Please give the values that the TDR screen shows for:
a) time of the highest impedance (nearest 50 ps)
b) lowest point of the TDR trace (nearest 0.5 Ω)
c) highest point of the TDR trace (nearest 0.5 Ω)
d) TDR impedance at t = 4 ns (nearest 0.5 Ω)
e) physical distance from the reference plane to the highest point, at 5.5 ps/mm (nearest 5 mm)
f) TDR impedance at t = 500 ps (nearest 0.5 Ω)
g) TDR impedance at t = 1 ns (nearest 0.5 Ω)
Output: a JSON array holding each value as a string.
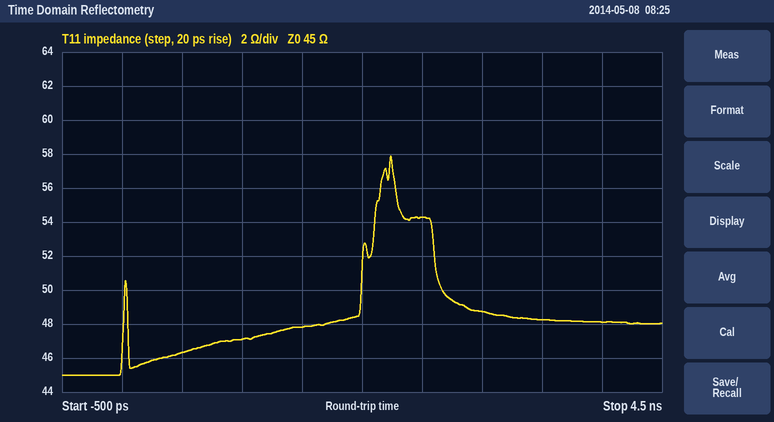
["2.25 ns", "45.0 Ω", "58.0 Ω", "48.0 Ω", "205 mm", "46.5 Ω", "47.0 Ω"]
